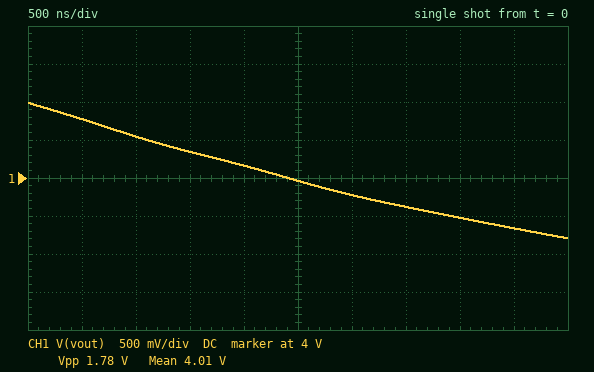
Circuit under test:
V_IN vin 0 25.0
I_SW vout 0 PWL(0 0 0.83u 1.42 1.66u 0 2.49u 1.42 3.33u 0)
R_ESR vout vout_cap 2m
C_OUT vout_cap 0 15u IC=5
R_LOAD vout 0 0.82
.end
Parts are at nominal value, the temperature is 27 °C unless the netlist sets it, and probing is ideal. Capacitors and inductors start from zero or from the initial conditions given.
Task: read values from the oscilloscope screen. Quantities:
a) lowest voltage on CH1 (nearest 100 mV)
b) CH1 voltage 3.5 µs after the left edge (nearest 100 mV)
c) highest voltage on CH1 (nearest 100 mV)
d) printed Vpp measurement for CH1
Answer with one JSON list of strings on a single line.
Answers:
["3.2 V", "3.6 V", "5.0 V", "1.78 V"]
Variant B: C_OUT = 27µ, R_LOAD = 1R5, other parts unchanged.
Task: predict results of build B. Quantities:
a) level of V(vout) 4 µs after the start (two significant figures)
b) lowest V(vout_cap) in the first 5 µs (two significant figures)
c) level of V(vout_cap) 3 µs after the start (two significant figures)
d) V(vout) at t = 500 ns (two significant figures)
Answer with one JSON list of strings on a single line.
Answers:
["4.4 V", "4.3 V", "4.6 V", "4.9 V"]
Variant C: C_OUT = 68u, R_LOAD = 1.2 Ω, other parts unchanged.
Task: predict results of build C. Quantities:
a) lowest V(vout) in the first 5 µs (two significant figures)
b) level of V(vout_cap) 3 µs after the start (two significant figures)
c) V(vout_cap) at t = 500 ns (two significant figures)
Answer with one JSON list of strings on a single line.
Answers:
["4.7 V", "4.8 V", "5.0 V"]
